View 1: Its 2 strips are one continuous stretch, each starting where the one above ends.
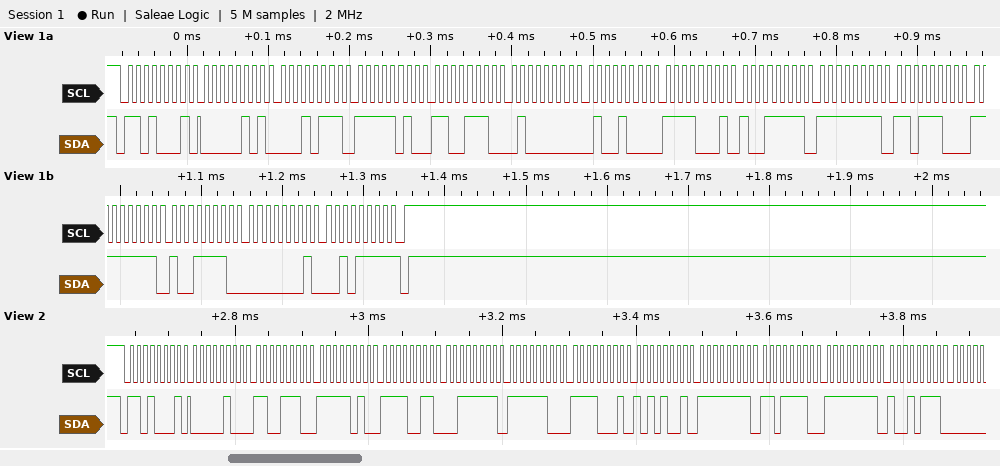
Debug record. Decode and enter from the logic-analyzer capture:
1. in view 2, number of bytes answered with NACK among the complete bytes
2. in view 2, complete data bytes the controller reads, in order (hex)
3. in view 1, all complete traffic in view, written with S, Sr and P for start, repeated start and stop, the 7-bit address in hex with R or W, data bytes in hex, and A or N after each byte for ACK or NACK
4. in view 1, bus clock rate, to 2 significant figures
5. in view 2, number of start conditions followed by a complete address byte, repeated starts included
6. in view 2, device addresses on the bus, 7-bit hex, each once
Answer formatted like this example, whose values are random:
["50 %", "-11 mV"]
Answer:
["0", "04 CE FA F3 3F FC F1 A9 FF DE FF 97", "S 68R A 05 A 17 A FA A CE A 40 A 48 A F1 A 9F A FF A DC A FF A 9E A 01 A 2F N P", "100 kHz", "1", "0x68"]
